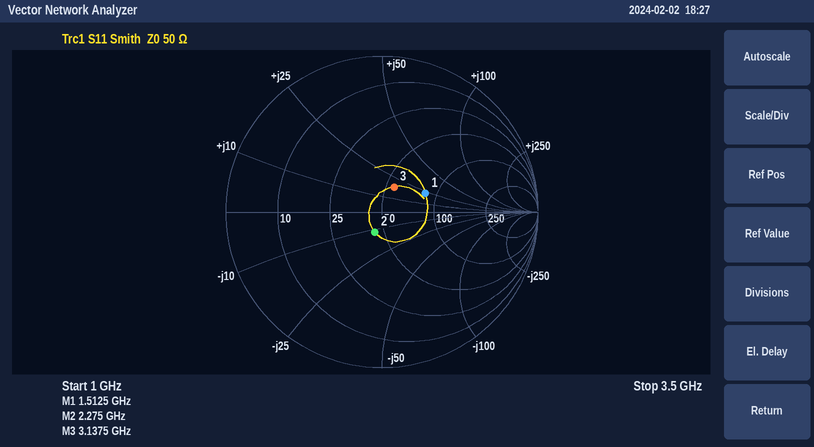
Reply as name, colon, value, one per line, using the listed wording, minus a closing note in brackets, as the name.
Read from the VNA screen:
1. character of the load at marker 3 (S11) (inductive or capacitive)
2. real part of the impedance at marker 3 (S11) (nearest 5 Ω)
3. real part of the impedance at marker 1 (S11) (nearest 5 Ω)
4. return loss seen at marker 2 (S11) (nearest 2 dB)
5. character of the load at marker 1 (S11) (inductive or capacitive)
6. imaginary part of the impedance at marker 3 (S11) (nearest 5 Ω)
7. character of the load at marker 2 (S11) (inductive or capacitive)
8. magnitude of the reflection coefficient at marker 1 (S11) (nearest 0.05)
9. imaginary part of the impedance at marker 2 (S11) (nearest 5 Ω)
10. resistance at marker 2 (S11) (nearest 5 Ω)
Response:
character of the load at marker 3 (S11): inductive
real part of the impedance at marker 3 (S11): 55 Ω
real part of the impedance at marker 1 (S11): 85 Ω
return loss seen at marker 2 (S11): 18 dB
character of the load at marker 1 (S11): inductive
imaginary part of the impedance at marker 3 (S11): +20 Ω
character of the load at marker 2 (S11): capacitive
magnitude of the reflection coefficient at marker 1 (S11): 0.30
imaginary part of the impedance at marker 2 (S11): -10 Ω
resistance at marker 2 (S11): 45 Ω
